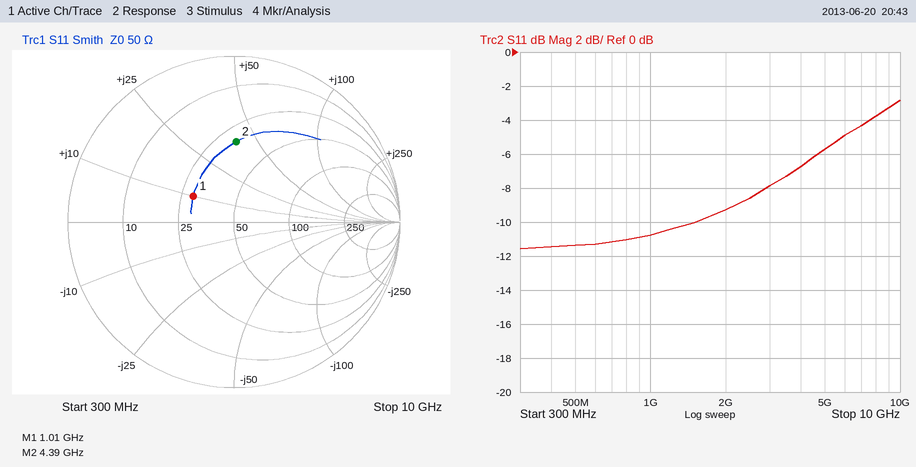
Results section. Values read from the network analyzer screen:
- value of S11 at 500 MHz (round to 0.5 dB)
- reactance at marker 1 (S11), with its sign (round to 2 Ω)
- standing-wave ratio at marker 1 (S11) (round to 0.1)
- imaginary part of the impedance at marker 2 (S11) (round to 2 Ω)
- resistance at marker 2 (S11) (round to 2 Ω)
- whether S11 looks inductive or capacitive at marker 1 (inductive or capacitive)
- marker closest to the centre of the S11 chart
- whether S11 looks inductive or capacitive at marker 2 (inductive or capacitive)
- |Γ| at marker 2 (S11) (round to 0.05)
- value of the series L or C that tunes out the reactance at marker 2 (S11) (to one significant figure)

-11.5 dB
+10 Ω
1.8
+40 Ω
32 Ω
inductive
marker 1
inductive
0.50
900 fF
